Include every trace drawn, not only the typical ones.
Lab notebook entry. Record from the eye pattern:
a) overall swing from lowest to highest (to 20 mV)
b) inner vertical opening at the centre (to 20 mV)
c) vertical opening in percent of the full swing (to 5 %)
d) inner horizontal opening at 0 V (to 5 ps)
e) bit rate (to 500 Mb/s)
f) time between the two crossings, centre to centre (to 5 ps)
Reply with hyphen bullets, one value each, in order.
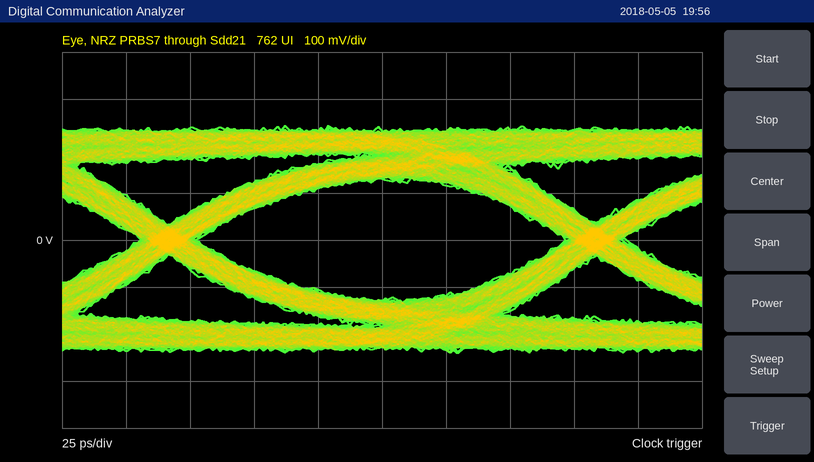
- 480 mV
- 260 mV
- 55 %
- 145 ps
- 6.0 Gb/s
- 165 ps
